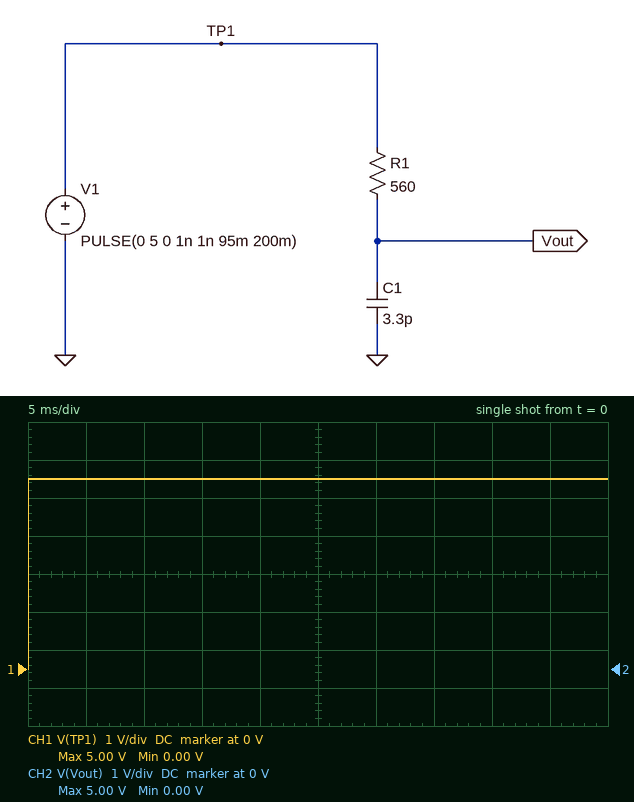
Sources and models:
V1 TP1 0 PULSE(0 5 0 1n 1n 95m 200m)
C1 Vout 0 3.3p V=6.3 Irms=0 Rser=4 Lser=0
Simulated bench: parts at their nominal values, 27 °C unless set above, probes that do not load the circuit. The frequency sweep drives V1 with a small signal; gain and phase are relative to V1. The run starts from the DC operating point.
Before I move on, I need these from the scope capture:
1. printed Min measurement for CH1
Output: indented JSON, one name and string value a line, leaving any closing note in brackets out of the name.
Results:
{
  "printed Min measurement for CH1": "0.00 V"
}
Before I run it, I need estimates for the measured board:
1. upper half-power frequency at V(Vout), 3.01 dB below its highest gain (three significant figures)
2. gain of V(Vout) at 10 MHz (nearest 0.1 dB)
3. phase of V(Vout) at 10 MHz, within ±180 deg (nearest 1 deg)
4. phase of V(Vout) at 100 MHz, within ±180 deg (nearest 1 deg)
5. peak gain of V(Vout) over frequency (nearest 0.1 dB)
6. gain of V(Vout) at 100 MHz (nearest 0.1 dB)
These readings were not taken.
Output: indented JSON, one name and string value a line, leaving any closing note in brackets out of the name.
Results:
{
  "upper half-power frequency at V(Vout), 3.01 dB below its highest gain": "85.5 MHz",
  "gain of V(Vout) at 10 MHz": "-0.1 dB",
  "phase of V(Vout) at 10 MHz, within ±180 deg": "-7 deg",
  "phase of V(Vout) at 100 MHz, within ±180 deg": "-49 deg",
  "peak gain of V(Vout) over frequency": "0 dB",
  "gain of V(Vout) at 100 MHz": "-3.7 dB"
}
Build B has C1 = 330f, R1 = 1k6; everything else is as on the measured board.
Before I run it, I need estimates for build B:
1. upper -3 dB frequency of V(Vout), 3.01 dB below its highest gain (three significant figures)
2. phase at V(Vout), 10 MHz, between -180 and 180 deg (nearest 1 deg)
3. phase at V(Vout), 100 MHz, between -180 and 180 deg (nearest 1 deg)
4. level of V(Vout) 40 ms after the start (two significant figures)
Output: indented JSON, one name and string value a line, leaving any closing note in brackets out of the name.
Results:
{
  "upper -3 dB frequency of V(Vout), 3.01 dB below its highest gain": "301 MHz",
  "phase at V(Vout), 10 MHz, between -180 and 180 deg": "-2 deg",
  "phase at V(Vout), 100 MHz, between -180 and 180 deg": "-18 deg",
  "level of V(Vout) 40 ms after the start": "5.0 V"
}
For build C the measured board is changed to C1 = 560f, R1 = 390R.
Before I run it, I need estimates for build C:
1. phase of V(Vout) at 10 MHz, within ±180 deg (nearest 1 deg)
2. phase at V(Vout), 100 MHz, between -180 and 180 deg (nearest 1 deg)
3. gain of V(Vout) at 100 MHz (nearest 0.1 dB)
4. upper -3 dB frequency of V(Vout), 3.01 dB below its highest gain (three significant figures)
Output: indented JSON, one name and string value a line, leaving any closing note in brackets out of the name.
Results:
{
  "phase of V(Vout) at 10 MHz, within ±180 deg": "-1 deg",
  "phase at V(Vout), 100 MHz, between -180 and 180 deg": "-8 deg",
  "gain of V(Vout) at 100 MHz": "-0.1 dB",
  "upper -3 dB frequency of V(Vout), 3.01 dB below its highest gain": "721 MHz"
}
